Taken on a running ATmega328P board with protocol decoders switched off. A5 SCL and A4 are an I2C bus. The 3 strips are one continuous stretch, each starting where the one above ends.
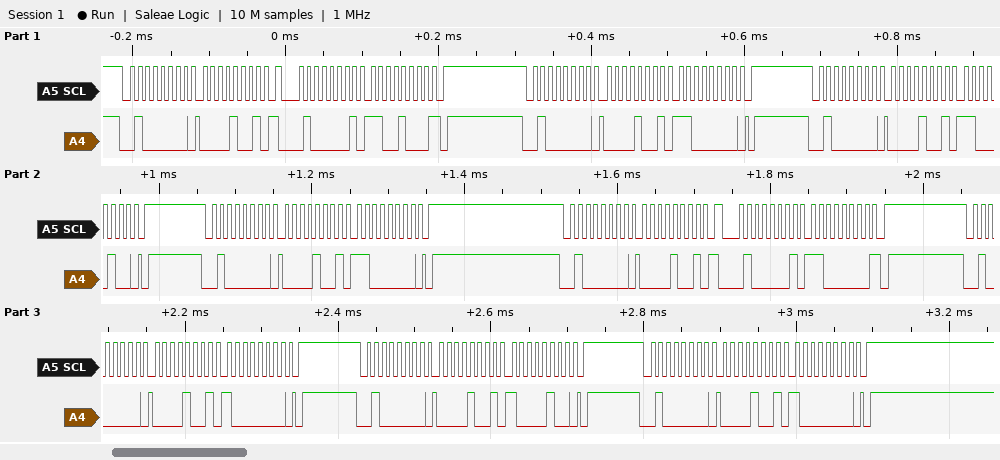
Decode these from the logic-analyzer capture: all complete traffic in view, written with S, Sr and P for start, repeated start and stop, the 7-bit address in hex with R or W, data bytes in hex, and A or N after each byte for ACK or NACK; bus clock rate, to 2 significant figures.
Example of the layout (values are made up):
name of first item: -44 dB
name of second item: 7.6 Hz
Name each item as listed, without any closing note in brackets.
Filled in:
all complete traffic in view, written with S, Sr and P for start, repeated start and stop, the 7-bit address in hex with R or W, data bytes in hex, and A or N after each byte for ACK or NACK: S 20W A 09 A Sr 20R A C8 N P S 20W A 09 A C0 A P S 20W A 09 A C4 A P S 20W A 09 A C0 A P S 20W A 09 A Sr 20R A C0 N P S 20W A 09 A 80 A P S 20W A 09 A 84 A P S 20W A 09 A 80 A P
bus clock rate, to 2 significant figures: 100 kHz
